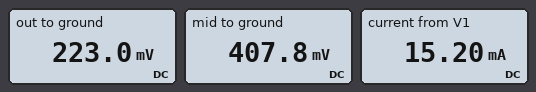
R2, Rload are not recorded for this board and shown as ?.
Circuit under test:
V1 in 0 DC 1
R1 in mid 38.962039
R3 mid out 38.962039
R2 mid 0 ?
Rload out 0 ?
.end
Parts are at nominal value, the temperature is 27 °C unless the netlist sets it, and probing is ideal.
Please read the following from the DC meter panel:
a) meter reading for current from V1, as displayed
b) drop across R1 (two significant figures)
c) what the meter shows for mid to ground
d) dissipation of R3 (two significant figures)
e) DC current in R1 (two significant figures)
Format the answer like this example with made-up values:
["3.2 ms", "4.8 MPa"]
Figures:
["15.20 mA", "590 mV", "407.8 mV", "880 µW", "15 mA"]
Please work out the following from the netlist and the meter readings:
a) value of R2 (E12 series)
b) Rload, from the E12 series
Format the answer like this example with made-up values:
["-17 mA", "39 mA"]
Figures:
["39 Ω", "47 Ω"]
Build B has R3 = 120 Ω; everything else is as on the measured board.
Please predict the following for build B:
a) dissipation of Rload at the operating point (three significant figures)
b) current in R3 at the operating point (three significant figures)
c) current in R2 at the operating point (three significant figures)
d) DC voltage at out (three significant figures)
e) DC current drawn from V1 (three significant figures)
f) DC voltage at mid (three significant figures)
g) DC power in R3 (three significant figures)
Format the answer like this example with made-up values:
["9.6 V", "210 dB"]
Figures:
["338 µW", "2.68 mA", "11.5 mA", "126 mV", "14.2 mA", "448 mV", "863 µW"]
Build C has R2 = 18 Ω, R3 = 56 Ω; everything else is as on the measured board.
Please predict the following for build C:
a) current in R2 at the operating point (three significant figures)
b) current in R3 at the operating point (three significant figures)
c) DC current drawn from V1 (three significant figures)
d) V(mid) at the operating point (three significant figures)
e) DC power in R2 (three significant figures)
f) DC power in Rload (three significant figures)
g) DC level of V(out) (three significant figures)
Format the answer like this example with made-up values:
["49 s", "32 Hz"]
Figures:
["15.7 mA", "2.74 mA", "18.4 mA", "282 mV", "4.43 mW", "353 µW", "129 mV"]
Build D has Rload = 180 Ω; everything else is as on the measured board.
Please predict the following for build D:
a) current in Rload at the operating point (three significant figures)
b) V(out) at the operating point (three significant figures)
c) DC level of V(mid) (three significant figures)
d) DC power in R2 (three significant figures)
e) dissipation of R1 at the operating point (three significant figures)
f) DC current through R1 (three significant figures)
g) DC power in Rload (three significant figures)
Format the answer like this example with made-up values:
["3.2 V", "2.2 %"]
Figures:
["2.10 mA", "378 mV", "459 mV", "5.41 mW", "7.50 mW", "13.9 mA", "792 µW"]
